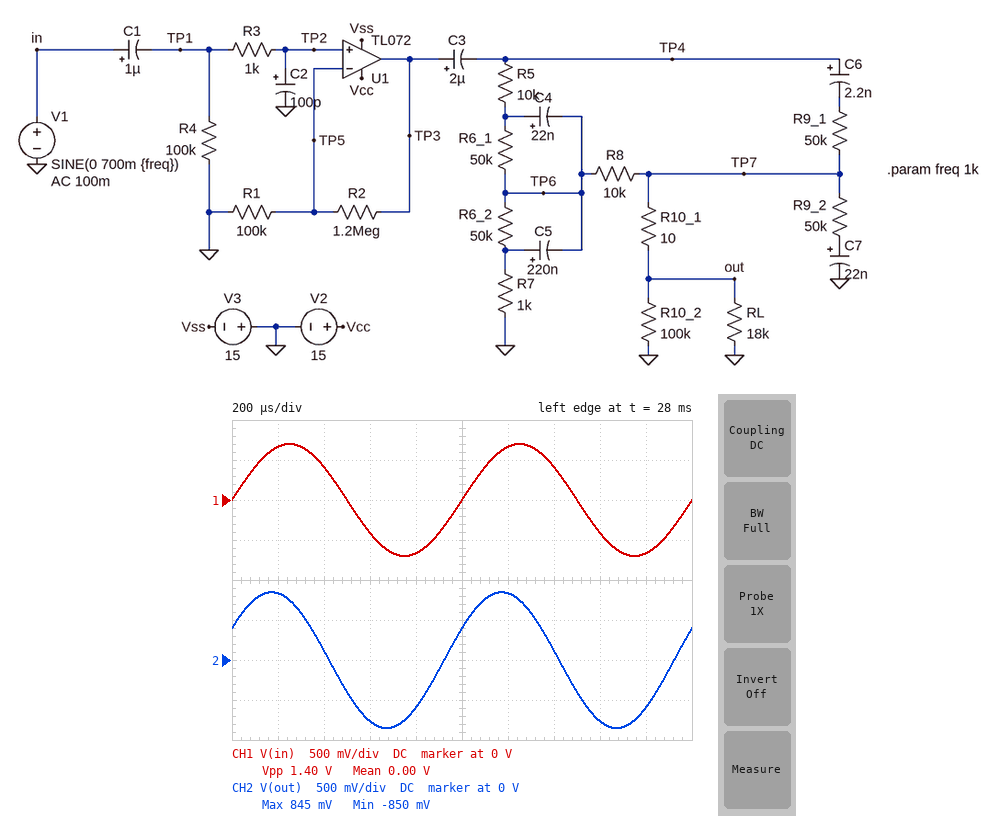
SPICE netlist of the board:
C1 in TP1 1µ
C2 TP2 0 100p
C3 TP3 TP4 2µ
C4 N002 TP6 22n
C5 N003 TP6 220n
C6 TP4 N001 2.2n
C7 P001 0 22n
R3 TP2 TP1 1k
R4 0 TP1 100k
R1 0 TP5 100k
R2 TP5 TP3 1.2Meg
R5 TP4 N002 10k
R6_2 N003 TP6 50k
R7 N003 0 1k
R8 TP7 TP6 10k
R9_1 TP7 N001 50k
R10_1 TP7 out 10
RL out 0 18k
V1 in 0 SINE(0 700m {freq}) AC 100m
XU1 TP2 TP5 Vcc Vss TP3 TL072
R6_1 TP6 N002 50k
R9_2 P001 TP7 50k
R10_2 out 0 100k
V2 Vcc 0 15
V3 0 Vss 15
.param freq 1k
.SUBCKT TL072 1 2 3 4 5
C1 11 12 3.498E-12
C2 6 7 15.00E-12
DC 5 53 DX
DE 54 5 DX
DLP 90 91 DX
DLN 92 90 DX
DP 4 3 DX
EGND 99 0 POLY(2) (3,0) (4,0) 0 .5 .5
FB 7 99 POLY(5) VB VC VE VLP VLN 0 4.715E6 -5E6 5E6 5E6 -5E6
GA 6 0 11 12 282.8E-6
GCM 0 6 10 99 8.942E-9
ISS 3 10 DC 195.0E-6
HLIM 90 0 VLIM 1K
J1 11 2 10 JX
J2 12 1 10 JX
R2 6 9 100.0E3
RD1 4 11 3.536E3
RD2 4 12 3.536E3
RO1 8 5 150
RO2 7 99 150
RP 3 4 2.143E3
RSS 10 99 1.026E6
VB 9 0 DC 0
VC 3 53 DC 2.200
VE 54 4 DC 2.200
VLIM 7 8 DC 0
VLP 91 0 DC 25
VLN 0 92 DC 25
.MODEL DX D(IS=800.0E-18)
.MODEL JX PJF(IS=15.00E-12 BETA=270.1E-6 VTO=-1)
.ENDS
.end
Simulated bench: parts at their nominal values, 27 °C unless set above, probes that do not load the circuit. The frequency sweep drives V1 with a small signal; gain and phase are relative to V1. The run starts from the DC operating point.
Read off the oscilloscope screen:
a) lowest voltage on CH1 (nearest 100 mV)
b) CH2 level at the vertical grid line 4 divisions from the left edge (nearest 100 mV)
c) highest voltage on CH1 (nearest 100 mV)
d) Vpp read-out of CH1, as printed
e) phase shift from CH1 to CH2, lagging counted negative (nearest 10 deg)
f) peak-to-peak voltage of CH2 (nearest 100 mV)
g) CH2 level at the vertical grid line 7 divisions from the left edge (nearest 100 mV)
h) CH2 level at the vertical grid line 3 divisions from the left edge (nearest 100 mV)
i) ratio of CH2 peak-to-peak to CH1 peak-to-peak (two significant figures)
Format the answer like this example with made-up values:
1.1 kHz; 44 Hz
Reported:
-700 mV; -600 mV; 700 mV; 1.40 V; 30 deg; 1.7 V; 100 mV; -800 mV; 1.2
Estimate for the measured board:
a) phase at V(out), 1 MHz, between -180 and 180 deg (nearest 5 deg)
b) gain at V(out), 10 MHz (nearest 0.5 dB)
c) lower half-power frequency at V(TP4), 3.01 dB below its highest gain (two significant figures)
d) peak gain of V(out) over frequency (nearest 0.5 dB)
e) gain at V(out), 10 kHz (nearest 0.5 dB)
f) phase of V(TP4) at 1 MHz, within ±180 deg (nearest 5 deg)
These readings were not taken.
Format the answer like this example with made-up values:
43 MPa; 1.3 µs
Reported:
-115 deg; -47.5 dB; 2.1 Hz; 5.5 dB; 5.5 dB; -115 deg
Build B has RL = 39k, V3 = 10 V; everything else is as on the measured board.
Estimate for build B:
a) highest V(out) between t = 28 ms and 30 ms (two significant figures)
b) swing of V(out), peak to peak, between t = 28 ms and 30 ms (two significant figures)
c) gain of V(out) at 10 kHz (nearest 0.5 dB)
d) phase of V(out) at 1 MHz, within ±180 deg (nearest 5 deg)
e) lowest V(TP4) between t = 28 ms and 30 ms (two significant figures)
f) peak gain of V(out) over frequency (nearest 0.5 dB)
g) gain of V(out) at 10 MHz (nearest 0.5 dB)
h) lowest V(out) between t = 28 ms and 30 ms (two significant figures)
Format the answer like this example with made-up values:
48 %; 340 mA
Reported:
1.0 V; 2.0 V; 7.0 dB; -115 deg; -8.4 V; 7.5 dB; -46.0 dB; -1.0 V
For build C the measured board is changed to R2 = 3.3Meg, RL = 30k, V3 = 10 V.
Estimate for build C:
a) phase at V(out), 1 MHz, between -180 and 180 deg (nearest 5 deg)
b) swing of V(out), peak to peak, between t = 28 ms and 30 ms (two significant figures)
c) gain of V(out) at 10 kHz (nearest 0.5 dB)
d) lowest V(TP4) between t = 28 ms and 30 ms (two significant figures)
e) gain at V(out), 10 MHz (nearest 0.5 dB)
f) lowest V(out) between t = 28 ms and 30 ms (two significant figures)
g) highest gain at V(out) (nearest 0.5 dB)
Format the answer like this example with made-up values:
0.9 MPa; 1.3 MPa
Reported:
-125 deg; 3.7 V; 14.5 dB; -8.8 V; -46.5 dB; -1.6 V; 15.0 dB
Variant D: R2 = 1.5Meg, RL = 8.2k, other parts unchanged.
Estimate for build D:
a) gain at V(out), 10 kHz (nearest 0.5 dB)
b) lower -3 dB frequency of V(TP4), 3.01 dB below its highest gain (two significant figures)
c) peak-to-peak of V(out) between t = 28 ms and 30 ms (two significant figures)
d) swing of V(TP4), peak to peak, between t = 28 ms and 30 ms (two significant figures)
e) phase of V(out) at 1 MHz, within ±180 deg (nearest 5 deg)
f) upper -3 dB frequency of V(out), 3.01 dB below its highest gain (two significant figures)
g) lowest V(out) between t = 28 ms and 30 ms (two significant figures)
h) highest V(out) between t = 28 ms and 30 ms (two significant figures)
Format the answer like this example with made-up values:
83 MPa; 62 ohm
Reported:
4.5 dB; 2.1 Hz; 1.5 V; 22 V; -120 deg; 220 kHz; -770 mV; 770 mV
